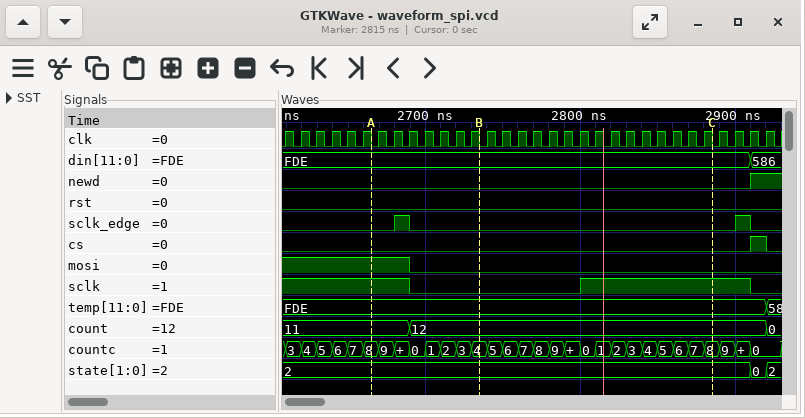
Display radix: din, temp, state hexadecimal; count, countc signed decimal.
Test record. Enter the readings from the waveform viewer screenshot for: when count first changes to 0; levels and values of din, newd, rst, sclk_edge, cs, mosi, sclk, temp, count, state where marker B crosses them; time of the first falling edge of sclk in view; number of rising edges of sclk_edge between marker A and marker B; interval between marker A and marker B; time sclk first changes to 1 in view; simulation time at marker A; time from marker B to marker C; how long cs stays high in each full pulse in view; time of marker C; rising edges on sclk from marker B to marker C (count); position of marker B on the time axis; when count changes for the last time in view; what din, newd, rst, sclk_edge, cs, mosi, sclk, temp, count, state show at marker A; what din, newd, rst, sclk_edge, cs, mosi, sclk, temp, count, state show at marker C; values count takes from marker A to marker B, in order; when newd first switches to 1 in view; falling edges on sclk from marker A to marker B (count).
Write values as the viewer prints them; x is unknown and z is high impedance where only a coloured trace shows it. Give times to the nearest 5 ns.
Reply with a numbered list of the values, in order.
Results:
1. 2920 ns
2. din=FDE, newd=0, rst=0, sclk_edge=0, cs=0, mosi=0, sclk=0, temp=FDE, count=12, state=2
3. 2690 ns
4. 1
5. 70 ns
6. 2800 ns
7. 2665 ns
8. 150 ns
9. 10 ns
10. 2885 ns
11. 1
12. 2735 ns
13. 2920 ns
14. din=FDE, newd=0, rst=0, sclk_edge=0, cs=0, mosi=1, sclk=1, temp=FDE, count=11, state=2
15. din=FDE, newd=0, rst=0, sclk_edge=0, cs=0, mosi=0, sclk=1, temp=FDE, count=12, state=2
16. 11, 12
17. 2910 ns
18. 1
